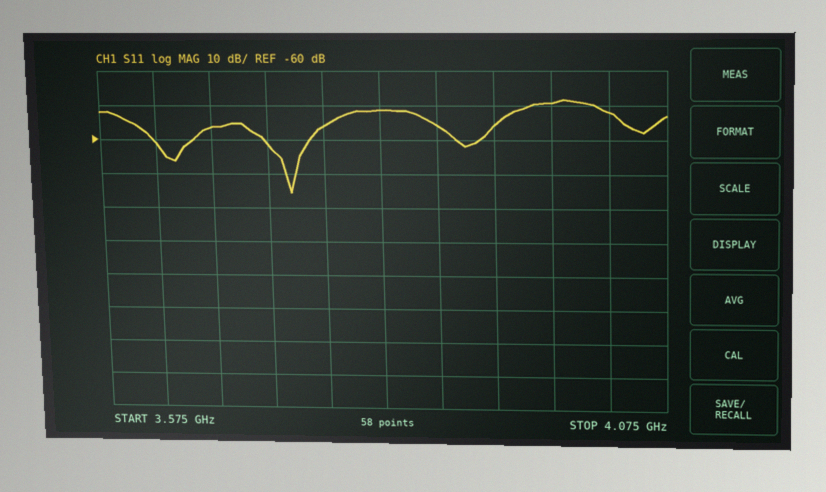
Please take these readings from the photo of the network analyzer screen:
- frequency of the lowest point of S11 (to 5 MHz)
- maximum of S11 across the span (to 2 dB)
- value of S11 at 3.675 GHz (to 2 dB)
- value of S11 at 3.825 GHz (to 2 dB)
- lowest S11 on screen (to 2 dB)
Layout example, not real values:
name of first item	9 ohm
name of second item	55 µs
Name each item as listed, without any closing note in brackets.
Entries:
frequency of the lowest point of S11	3.745 GHz
maximum of S11 across the span	-48 dB
value of S11 at 3.675 GHz	-56 dB
value of S11 at 3.825 GHz	-52 dB
lowest S11 on screen	-76 dB
